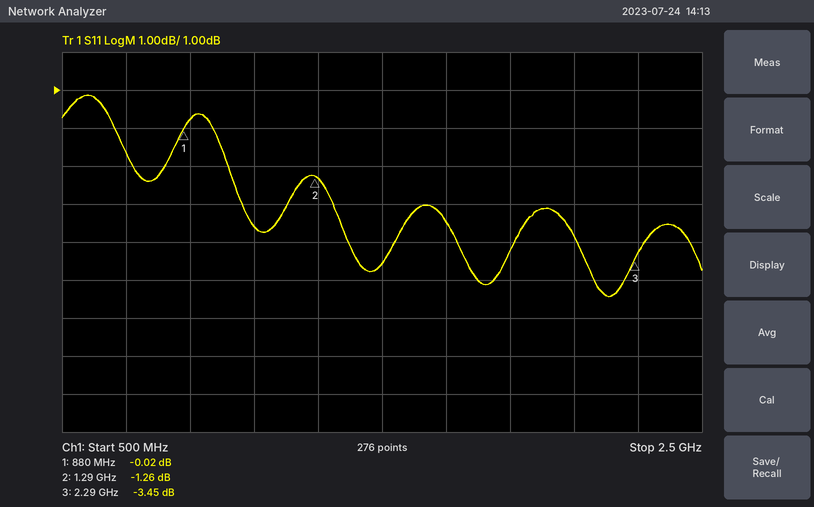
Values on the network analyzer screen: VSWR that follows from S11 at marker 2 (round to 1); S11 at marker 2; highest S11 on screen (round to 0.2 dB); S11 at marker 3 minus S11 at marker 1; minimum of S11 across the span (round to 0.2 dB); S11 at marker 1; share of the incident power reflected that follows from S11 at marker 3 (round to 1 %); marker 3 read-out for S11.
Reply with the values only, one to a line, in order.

14
-1.26 dB
0.8 dB
-3.43 dB
-4.4 dB
-0.02 dB
45 %
-3.45 dB
